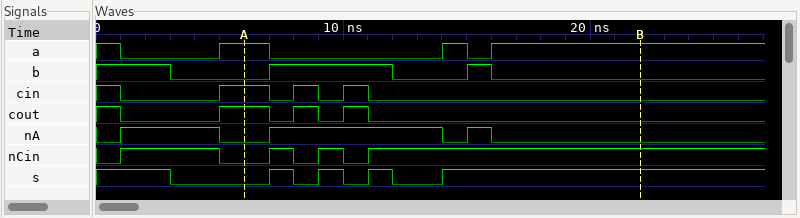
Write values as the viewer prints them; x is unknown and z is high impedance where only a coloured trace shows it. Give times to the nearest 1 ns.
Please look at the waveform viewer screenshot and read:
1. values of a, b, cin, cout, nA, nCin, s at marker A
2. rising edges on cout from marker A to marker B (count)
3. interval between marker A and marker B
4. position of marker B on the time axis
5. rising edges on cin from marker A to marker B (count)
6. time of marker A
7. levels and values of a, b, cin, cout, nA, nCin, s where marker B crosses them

a=1, b=0, cin=1, cout=1, nA=0, nCin=0, s=0
2
16 ns
22 ns
2
6 ns
a=1, b=0, cin=0, cout=0, nA=0, nCin=1, s=1
